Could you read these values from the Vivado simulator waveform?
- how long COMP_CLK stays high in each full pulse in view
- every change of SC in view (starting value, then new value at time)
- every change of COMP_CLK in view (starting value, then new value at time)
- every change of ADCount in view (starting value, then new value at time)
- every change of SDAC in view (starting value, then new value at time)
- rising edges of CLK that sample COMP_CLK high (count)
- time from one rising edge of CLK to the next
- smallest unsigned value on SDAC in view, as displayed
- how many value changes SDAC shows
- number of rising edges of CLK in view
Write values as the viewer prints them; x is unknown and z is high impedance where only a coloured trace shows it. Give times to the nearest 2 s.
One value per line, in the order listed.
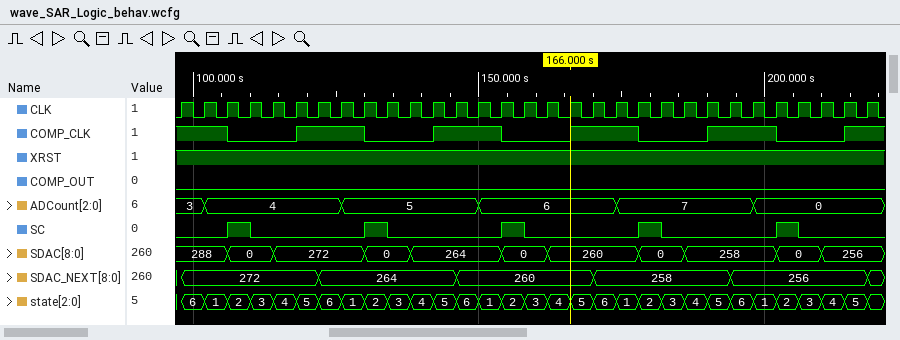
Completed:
12 s, 12 s, 12 s, 12 s
0, 1 at 106 s, 0 at 110 s, 1 at 130 s, 0 at 134 s, 1 at 154 s, 0 at 158 s, 1 at 178 s, 0 at 182 s, 1 at 202 s, 0 at 206 s
1, 0 at 106 s, 1 at 118 s, 0 at 130 s, 1 at 142 s, 0 at 154 s, 1 at 166 s, 0 at 178 s, 1 at 190 s, 0 at 202 s, 1 at 214 s
3, 4 at 102 s, 5 at 126 s, 6 at 150 s, 7 at 174 s, 0 at 198 s
288, 0 at 106 s, 272 at 114 s, 0 at 130 s, 264 at 138 s, 0 at 154 s, 260 at 162 s, 0 at 178 s, 258 at 186 s, 0 at 202 s, 256 at 210 s
16
4 s
0
10
31
